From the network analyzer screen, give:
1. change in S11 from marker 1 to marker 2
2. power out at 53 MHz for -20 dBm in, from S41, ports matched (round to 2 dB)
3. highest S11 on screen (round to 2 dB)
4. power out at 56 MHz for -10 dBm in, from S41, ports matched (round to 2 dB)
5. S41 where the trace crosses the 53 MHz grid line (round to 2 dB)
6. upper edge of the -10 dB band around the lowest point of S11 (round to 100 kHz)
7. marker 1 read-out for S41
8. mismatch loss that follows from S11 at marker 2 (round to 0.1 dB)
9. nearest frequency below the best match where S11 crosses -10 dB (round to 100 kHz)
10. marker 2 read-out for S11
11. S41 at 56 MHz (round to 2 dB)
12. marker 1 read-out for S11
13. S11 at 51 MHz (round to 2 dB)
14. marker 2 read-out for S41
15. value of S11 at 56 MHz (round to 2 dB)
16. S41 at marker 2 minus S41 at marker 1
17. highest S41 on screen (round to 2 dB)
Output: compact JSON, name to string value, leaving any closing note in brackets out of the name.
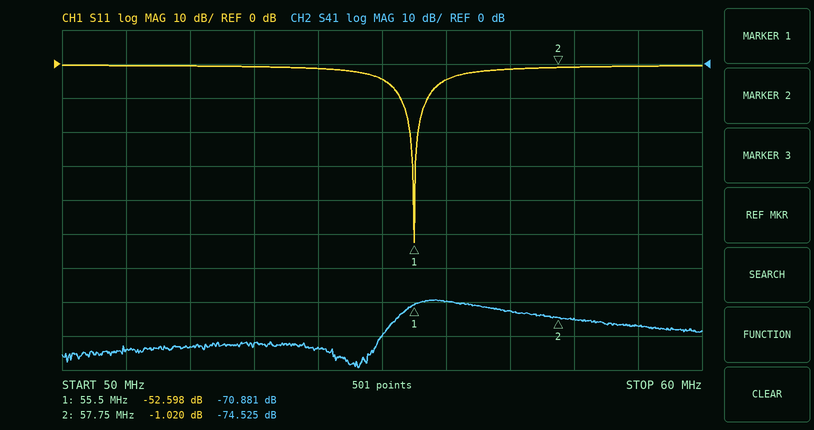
{"change in S11 from marker 1 to marker 2": "51.578 dB", "power out at 53 MHz for -20 dBm in, from S41, ports matched": "-102 dBm", "highest S11 on screen": "0 dB", "power out at 56 MHz for -10 dBm in, from S41, ports matched": "-80 dBm", "S41 where the trace crosses the 53 MHz grid line": "-82 dB", "upper edge of the -10 dB band around the lowest point of S11": "55.7 MHz", "marker 1 read-out for S41": "-70.881 dB", "mismatch loss that follows from S11 at marker 2": "6.8 dB", "nearest frequency below the best match where S11 crosses -10 dB": "55.3 MHz", "marker 2 read-out for S11": "-1.020 dB", "S41 at 56 MHz": "-70 dB", "marker 1 read-out for S11": "-52.598 dB", "S11 at 51 MHz": "0 dB", "marker 2 read-out for S41": "-74.525 dB", "value of S11 at 56 MHz": "-4 dB", "S41 at marker 2 minus S41 at marker 1": "-3.644 dB", "highest S41 on screen": "-70 dB"}
